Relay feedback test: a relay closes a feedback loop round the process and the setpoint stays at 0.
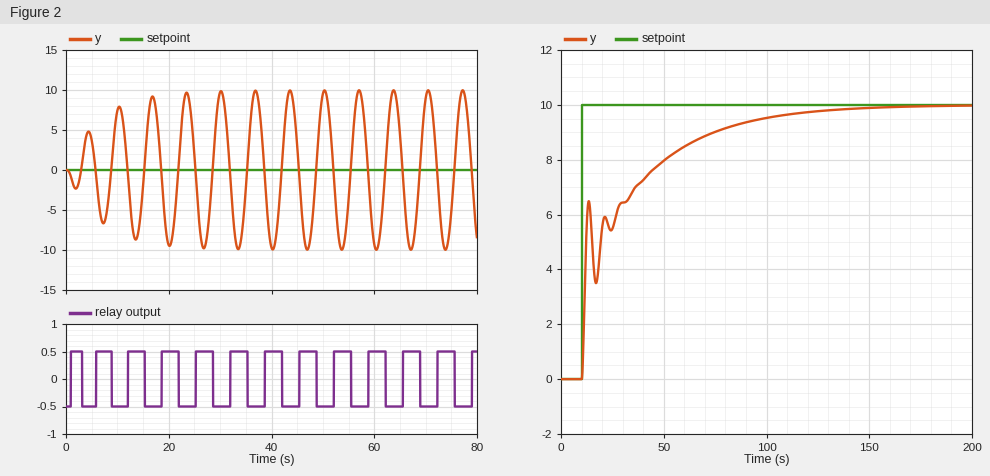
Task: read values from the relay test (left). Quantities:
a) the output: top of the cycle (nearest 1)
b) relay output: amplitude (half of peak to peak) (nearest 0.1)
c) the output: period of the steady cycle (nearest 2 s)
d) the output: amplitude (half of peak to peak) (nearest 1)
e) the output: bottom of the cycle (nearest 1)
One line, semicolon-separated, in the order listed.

10; 0.5; 6 s; 10; -10
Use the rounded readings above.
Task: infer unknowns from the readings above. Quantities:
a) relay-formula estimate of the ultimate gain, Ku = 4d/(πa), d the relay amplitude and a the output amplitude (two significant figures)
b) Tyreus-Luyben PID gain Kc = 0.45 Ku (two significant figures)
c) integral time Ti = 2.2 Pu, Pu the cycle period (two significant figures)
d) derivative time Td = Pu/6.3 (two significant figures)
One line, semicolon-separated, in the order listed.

0.064; 0.029; 13 s; 0.95 s
